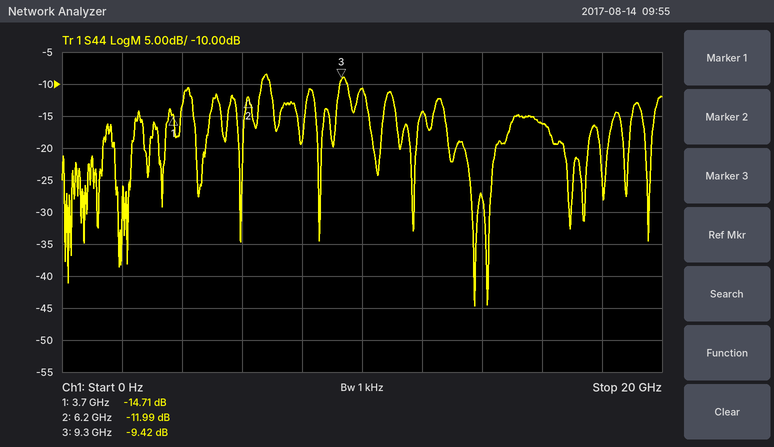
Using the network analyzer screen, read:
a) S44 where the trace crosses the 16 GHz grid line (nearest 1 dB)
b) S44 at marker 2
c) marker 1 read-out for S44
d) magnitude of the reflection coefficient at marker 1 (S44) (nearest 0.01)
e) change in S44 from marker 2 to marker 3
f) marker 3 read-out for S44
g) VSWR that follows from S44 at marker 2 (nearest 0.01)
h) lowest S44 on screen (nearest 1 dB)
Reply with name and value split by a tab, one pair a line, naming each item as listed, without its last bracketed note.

S44 where the trace crosses the 16 GHz grid line	-16 dB
S44 at marker 2	-11.99 dB
marker 1 read-out for S44	-14.71 dB
magnitude of the reflection coefficient at marker 1 (S44)	0.18
change in S44 from marker 2 to marker 3	2.57 dB
marker 3 read-out for S44	-9.42 dB
VSWR that follows from S44 at marker 2	1.67
lowest S44 on screen	-45 dB
